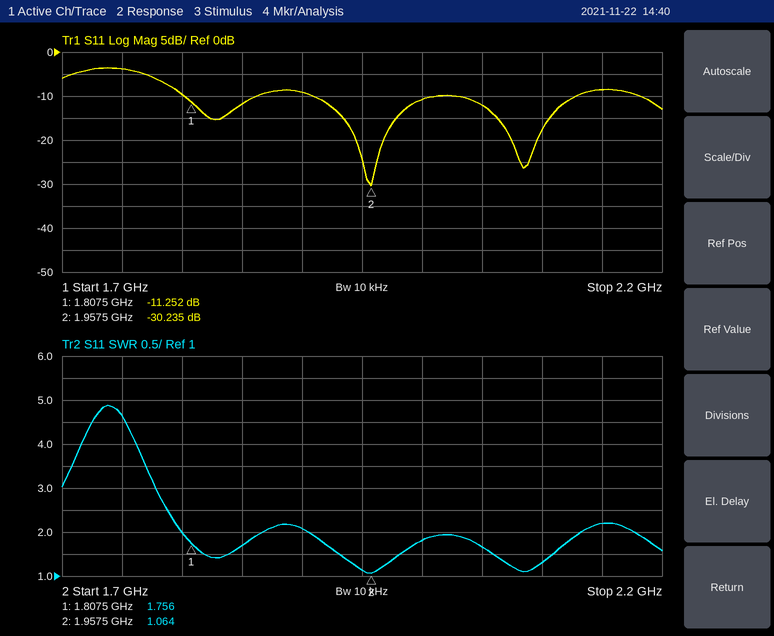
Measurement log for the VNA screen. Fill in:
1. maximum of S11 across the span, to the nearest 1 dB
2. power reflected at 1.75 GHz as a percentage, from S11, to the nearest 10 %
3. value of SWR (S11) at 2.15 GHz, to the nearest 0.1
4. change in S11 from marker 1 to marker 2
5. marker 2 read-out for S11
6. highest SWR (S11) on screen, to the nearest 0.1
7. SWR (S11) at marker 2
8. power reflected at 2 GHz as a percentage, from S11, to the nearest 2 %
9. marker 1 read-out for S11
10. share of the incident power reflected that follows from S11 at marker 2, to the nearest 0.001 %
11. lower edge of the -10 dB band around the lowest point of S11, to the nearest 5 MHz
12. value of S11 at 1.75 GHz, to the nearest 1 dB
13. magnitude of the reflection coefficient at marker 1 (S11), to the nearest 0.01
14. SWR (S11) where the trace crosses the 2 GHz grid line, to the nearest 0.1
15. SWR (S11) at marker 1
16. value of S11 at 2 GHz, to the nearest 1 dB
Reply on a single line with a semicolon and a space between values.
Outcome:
-4 dB; 40 %; 2.2; -18.983 dB; -30.235 dB; 4.9; 1.064; 8 %; -11.252 dB; 0.095 %; 1.910 GHz; -4 dB; 0.27; 1.8; 1.756; -11 dB
